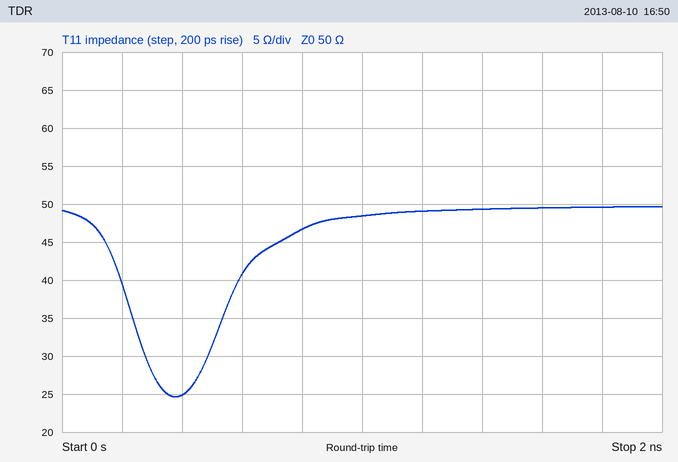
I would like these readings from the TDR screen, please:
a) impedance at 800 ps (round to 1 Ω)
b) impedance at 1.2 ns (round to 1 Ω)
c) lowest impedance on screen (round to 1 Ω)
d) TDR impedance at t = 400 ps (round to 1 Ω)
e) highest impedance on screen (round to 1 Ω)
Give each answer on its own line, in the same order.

47 Ω
49 Ω
25 Ω
25 Ω
50 Ω
